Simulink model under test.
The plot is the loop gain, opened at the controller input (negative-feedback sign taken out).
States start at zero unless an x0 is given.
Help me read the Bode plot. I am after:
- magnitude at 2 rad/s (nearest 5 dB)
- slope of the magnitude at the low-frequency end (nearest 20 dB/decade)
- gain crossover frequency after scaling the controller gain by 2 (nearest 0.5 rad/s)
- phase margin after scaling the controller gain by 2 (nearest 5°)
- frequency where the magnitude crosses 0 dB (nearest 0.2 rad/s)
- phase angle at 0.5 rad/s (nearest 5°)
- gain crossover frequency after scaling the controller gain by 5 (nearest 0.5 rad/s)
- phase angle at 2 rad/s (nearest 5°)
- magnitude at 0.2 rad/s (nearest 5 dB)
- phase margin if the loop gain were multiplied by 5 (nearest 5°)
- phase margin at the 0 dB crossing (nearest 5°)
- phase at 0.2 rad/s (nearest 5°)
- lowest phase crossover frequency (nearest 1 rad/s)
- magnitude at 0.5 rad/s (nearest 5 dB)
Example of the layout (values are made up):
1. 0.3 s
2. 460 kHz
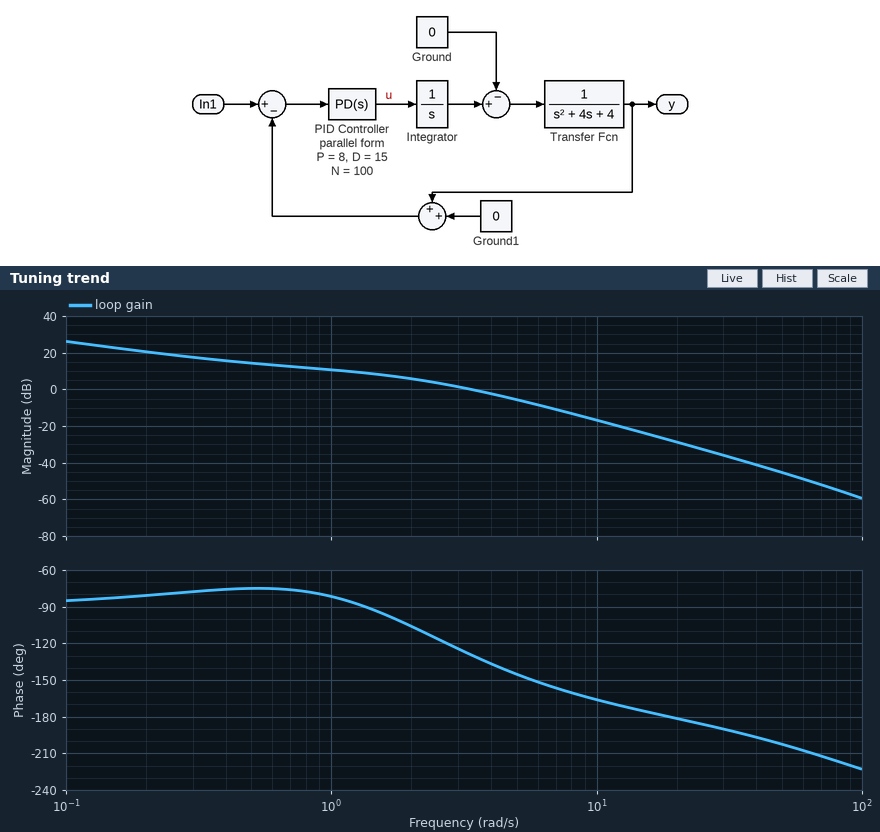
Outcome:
1. 5 dB
2. -20 dB/decade
3. 5.0 rad/s
4. 35°
5. 3.4 rad/s
6. -75°
7. 8.5 rad/s
8. -105°
9. 20 dB
10. 20°
11. 50°
12. -80°
13. 19 rad/s
14. 15 dB
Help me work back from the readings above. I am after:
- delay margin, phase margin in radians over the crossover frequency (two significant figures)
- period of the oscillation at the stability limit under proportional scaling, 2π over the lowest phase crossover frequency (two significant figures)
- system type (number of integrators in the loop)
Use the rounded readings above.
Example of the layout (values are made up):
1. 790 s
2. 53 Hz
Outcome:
1. 0.26 s
2. 0.33 s
3. 1
